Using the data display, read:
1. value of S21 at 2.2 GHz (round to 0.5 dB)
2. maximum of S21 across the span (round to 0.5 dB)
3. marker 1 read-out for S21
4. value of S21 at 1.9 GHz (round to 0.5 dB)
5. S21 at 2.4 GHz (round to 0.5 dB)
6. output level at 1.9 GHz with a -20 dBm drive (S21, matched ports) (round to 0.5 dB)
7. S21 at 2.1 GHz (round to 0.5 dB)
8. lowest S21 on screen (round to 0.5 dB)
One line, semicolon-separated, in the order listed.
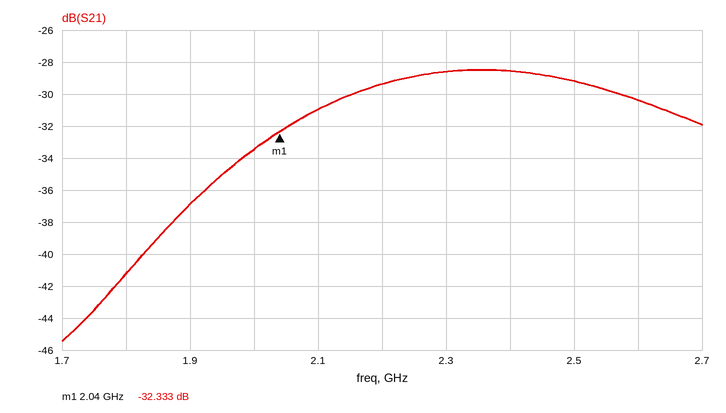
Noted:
-29.5 dB; -28.5 dB; -32.333 dB; -37.0 dB; -28.5 dB; -57.0 dBm; -31.0 dB; -45.5 dB
